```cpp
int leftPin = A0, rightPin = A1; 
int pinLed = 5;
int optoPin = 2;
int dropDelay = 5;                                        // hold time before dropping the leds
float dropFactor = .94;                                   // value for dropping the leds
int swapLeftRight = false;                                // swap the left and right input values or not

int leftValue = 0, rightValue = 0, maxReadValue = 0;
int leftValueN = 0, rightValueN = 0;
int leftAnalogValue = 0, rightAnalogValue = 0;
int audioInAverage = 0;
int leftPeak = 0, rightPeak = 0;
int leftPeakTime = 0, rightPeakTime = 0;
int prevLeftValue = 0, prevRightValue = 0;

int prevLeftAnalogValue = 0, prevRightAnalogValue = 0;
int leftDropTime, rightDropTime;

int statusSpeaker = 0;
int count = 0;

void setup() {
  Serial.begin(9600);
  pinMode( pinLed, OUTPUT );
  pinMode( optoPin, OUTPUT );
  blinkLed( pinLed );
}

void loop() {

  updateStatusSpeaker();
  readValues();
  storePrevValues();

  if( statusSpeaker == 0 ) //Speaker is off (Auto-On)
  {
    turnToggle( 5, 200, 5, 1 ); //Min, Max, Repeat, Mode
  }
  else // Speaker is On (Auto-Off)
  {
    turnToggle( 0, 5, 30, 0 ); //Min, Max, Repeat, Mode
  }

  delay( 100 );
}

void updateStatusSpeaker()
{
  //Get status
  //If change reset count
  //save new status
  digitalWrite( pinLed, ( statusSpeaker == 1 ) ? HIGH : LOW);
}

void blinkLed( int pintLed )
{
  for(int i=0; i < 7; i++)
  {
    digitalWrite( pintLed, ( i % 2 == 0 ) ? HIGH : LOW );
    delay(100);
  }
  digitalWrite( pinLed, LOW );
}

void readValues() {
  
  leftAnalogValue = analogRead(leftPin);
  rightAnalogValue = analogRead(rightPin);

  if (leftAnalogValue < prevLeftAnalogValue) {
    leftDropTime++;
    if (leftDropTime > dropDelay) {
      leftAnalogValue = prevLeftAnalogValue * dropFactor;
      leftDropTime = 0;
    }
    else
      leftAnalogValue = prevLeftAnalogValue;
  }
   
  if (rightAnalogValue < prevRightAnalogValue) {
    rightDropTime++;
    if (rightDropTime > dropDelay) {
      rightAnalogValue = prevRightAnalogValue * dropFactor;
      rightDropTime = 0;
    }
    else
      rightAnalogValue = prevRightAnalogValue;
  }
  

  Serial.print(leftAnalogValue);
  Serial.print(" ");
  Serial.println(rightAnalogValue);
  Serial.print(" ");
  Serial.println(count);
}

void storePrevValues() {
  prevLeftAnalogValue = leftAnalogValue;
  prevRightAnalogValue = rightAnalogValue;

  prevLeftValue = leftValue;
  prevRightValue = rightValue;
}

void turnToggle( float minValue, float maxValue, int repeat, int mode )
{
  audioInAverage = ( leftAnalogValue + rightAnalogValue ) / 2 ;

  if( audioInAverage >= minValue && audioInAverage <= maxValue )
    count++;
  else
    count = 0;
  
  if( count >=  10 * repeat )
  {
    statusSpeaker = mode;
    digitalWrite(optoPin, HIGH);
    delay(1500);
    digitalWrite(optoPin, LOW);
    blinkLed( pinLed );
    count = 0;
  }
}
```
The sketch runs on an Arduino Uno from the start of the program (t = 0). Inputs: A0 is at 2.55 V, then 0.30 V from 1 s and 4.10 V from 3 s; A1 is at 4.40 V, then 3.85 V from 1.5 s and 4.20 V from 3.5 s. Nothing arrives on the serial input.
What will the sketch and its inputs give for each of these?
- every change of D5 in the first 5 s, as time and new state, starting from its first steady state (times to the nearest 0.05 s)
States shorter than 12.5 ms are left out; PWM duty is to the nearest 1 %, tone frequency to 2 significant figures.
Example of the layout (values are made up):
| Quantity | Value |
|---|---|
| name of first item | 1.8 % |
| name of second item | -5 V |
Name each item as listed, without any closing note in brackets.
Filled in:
| Quantity | Value |
|---|---|
| every change of D5 in the first 5 s, as time and new state, starting from its first steady state | 0 s high; 0.1 s low; 0.2 s high; 0.3 s low; 0.4 s high; 0.5 s low; 0.6 s high; 0.7 s low |
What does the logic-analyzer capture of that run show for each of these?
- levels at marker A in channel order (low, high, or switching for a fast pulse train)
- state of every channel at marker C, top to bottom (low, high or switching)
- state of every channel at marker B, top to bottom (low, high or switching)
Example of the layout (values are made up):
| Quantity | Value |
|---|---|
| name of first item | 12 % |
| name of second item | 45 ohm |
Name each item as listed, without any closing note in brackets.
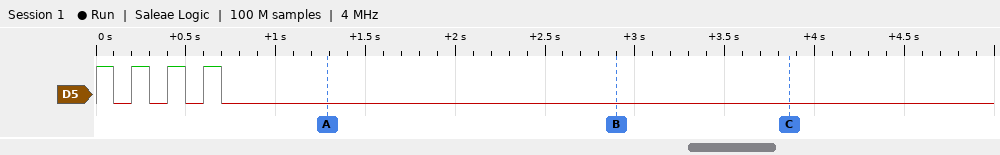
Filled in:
| Quantity | Value |
|---|---|
| levels at marker A in channel order | D5 low |
| state of every channel at marker C, top to bottom | D5 low |
| state of every channel at marker B, top to bottom | D5 low |
